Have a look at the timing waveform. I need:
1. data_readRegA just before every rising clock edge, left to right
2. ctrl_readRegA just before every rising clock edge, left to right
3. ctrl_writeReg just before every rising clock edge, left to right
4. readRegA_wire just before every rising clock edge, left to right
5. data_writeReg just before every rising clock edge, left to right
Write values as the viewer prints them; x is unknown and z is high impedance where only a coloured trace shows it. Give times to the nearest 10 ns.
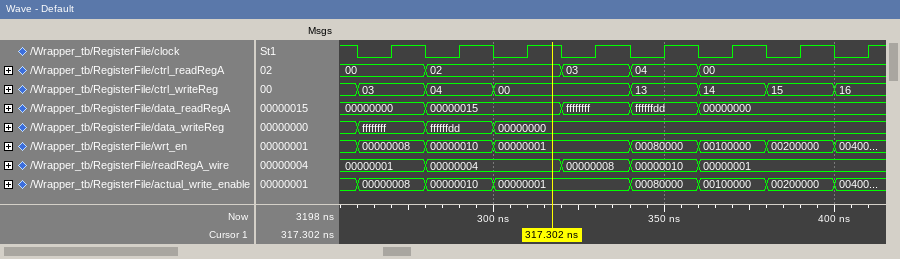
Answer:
00000000, 00000015, 00000015, ffffffff, ffffffdd, 00000000, 00000000, 00000000
00, 02, 02, 03, 04, 00, 00, 00
03, 04, 00, 00, 13, 14, 15, 16
00000001, 00000004, 00000004, 00000008, 00000010, 00000001, 00000001, 00000001
ffffffff, ffffffdd, 00000000, 00000000, 00000000, 00000000, 00000000, 00000000
